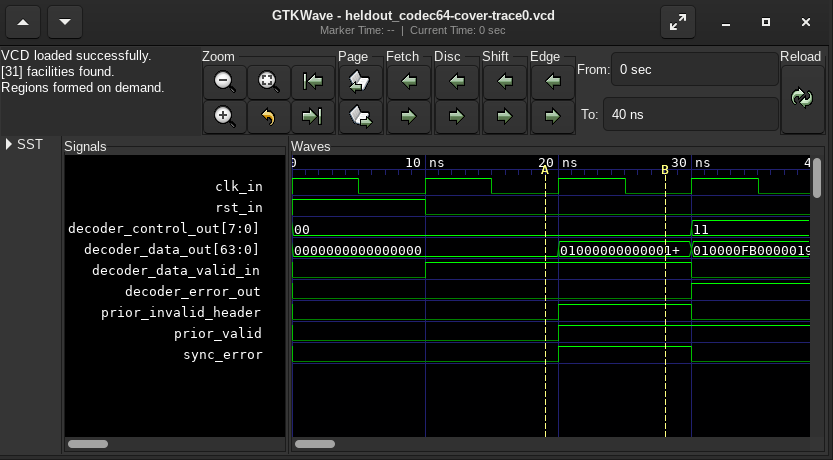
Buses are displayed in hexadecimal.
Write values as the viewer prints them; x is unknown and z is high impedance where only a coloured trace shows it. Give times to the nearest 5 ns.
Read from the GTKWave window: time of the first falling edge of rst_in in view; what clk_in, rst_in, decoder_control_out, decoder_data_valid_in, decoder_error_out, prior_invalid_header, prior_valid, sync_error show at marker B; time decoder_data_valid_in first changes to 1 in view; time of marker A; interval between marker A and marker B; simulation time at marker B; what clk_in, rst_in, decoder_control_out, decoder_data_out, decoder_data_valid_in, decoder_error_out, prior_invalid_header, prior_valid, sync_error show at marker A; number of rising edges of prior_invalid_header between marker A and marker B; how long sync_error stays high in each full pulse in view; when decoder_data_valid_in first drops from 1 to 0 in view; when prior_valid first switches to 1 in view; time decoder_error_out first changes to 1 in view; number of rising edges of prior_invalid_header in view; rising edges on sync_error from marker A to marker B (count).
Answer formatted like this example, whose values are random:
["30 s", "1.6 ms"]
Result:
["10 ns", "clk_in=0, rst_in=0, decoder_control_out=00, decoder_data_valid_in=1, decoder_error_out=0, prior_invalid_header=1, prior_valid=1, sync_error=1", "10 ns", "20 ns", "10 ns", "30 ns", "clk_in=0, rst_in=0, decoder_control_out=00, decoder_data_out=0000000000000000, decoder_data_valid_in=1, decoder_error_out=0, prior_invalid_header=0, prior_valid=0, sync_error=0", "1", "10 ns", "30 ns", "20 ns", "30 ns", "1", "1"]
